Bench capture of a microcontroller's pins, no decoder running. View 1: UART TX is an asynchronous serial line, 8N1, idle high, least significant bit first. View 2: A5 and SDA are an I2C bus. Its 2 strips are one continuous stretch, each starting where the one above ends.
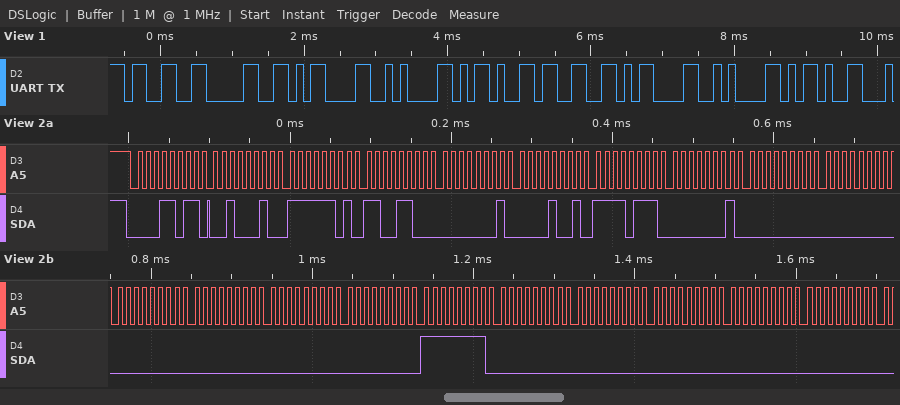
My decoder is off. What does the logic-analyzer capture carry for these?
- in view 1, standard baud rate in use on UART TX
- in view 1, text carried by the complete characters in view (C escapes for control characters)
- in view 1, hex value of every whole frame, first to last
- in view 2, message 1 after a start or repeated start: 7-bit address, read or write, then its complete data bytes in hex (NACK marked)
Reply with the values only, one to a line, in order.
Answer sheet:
9600 baud
"30\r\n-3\r\n-"
0x33 0x30 0x0D 0x0A 0x2D 0x33 0x0D 0x0A 0x2D
0x0D read: 22 FD CC 01 09 F7 01 00 00 00 00 00 00 FF 00 00 00 00 00
